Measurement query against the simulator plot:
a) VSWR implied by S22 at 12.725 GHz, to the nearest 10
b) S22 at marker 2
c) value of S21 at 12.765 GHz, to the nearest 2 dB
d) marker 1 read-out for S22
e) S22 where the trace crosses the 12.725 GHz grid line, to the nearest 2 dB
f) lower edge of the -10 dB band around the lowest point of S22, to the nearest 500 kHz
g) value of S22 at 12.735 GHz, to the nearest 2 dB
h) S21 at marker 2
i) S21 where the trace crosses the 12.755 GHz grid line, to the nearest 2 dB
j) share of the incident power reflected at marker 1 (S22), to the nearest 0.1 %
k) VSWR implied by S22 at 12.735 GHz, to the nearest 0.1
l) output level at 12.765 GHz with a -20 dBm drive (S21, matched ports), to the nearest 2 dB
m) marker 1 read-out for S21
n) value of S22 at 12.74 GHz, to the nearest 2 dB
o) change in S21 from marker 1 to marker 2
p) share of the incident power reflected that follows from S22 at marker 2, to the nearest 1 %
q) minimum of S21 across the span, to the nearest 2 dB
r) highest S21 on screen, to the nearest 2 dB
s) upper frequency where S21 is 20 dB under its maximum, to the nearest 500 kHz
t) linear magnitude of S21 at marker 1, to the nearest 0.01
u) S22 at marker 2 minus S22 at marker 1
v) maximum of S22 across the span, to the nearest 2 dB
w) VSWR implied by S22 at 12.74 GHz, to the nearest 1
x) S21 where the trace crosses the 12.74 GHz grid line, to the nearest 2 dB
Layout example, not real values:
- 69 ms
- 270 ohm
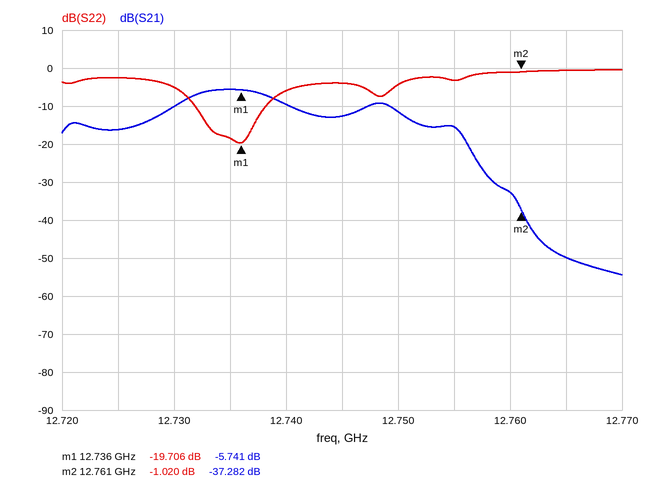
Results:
- 10
- -1.020 dB
- -50 dB
- -19.706 dB
- -2 dB
- 12.7320 GHz
- -18 dB
- -37.282 dB
- -16 dB
- 1.1 %
- 1.3
- -70 dBm
- -5.741 dB
- -6 dB
- -31.541 dB
- 79 %
- -54 dB
- -6 dB
- 12.7575 GHz
- 0.52
- 18.686 dB
- 0 dB
- 3
- -10 dB
